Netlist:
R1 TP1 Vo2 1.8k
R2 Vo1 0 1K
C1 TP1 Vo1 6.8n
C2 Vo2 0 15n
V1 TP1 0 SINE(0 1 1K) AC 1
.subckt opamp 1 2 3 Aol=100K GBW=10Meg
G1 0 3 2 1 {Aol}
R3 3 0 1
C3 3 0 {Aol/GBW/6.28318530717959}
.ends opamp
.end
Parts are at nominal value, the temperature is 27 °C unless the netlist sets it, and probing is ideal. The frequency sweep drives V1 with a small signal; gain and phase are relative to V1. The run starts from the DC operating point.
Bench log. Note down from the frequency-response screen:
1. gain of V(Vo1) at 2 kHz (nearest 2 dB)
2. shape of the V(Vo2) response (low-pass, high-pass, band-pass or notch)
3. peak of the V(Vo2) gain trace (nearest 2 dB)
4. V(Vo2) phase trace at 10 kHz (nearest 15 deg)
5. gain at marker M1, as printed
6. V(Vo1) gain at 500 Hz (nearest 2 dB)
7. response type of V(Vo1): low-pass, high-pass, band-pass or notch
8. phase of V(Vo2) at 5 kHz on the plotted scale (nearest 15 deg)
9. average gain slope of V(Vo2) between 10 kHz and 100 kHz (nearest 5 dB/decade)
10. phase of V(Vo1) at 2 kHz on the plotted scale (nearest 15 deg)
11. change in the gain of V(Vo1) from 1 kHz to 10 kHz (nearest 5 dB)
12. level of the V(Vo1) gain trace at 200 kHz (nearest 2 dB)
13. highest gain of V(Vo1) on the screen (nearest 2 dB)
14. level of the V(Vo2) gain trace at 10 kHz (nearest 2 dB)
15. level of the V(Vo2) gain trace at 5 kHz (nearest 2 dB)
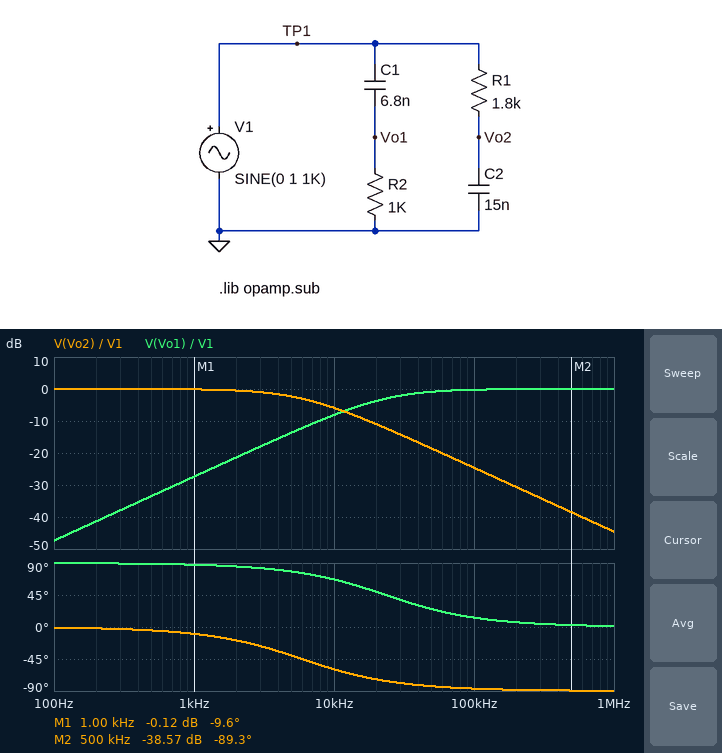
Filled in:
-22 dB
low-pass
0 dB
-60 deg
-0.12 dB
-34 dB
high-pass
-45 deg
-20 dB/decade
90 deg
20 dB
0 dB
0 dB
-6 dB
-2 dB
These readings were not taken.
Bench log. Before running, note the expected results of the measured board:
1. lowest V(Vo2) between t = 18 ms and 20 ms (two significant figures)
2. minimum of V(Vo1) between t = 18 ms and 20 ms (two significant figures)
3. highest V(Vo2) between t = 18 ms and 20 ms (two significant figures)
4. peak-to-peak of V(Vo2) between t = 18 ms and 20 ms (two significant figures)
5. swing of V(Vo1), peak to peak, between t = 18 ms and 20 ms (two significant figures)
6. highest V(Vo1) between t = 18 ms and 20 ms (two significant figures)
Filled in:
-990 mV
-43 mV
990 mV
2.0 V
85 mV
43 mV
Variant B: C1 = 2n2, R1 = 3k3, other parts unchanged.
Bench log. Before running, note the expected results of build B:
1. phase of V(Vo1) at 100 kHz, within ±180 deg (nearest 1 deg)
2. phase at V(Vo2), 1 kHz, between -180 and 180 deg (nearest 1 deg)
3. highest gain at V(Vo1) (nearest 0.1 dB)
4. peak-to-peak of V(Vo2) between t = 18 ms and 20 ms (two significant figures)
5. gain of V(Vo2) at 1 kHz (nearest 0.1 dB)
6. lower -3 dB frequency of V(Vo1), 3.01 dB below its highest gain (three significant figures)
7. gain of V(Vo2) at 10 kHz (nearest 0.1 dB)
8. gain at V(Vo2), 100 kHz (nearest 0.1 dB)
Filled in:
36 deg
-17 deg
0 dB
1.9 V
-0.4 dB
72.3 kHz
-10.3 dB
-29.9 dB
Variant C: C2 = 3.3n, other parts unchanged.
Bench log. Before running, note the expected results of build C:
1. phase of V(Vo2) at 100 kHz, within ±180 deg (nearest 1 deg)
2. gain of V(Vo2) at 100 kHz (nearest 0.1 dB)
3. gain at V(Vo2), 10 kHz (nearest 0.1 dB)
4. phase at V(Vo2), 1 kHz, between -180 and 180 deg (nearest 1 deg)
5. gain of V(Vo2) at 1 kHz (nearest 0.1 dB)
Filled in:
-75 deg
-11.7 dB
-0.6 dB
-2 deg
0 dB
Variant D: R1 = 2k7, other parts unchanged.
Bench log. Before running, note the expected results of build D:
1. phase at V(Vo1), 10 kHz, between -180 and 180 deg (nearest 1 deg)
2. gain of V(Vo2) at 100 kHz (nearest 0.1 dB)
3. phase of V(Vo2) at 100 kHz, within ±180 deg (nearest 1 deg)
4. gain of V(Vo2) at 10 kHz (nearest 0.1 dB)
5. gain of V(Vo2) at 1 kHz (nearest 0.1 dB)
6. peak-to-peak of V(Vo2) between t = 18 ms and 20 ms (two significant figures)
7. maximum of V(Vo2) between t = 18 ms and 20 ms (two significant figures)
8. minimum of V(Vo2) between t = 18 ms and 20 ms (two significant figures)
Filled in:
67 deg
-28.1 dB
-88 deg
-8.7 dB
-0.3 dB
1.9 V
970 mV
-970 mV
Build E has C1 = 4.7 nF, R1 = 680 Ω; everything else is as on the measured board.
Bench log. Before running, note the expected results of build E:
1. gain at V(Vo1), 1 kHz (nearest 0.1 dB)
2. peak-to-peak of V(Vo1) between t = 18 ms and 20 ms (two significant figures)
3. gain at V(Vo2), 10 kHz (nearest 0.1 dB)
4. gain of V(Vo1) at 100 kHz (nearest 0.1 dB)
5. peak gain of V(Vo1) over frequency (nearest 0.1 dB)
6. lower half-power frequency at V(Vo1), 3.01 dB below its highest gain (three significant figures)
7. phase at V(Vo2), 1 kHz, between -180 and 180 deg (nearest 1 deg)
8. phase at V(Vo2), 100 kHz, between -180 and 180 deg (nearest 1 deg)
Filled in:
-30.6 dB
59 mV
-1.5 dB
-0.5 dB
0 dB
33.9 kHz
-4 deg
-81 deg
